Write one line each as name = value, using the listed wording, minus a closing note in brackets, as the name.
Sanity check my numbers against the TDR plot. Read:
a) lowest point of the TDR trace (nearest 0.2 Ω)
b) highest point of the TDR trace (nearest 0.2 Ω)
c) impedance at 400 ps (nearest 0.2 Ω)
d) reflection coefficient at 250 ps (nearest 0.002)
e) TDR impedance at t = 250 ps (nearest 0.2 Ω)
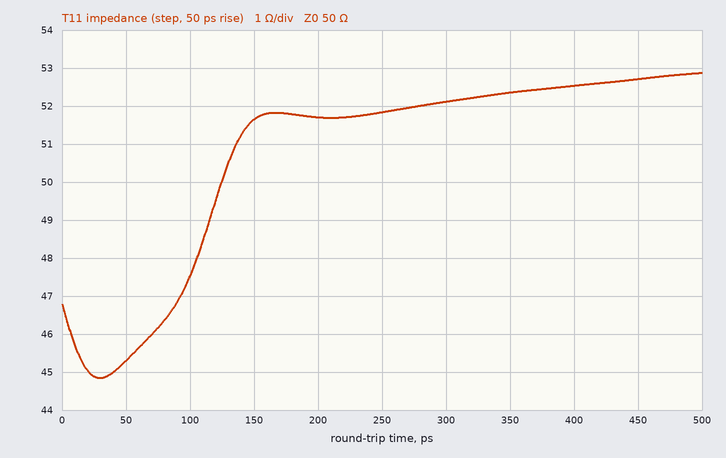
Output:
lowest point of the TDR trace = 44.8 Ω
highest point of the TDR trace = 52.8 Ω
impedance at 400 ps = 52.6 Ω
reflection coefficient at 250 ps = +0.018
TDR impedance at t = 250 ps = 51.8 Ω
